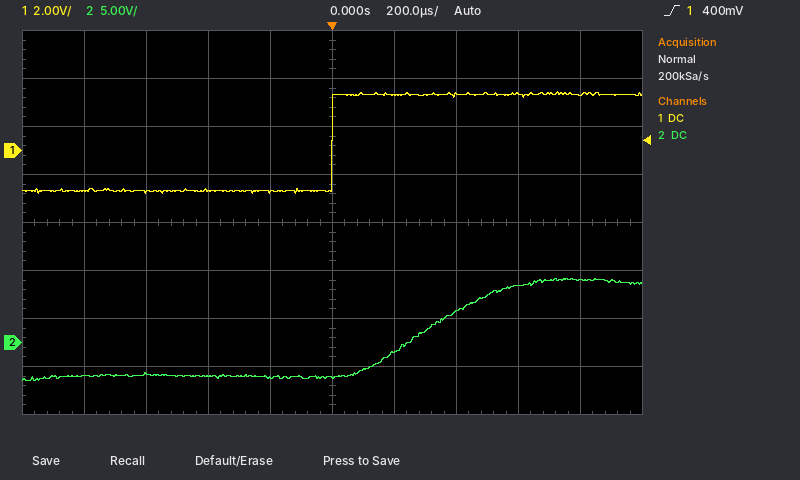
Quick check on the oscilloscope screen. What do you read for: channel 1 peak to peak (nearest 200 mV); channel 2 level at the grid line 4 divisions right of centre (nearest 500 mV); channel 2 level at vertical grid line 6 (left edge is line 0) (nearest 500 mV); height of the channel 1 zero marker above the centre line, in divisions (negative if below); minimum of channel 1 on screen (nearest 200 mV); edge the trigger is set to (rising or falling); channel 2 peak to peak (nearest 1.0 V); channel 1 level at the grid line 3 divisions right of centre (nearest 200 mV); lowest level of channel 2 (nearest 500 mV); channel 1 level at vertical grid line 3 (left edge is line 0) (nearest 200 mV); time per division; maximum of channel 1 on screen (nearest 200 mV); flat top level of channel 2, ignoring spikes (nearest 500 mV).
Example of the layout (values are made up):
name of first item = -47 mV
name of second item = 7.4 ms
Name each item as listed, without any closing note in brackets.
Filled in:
channel 1 peak to peak = 4.2 V
channel 2 level at the grid line 4 divisions right of centre = 6.5 V
channel 2 level at vertical grid line 6 (left edge is line 0) = -1.0 V
height of the channel 1 zero marker above the centre line, in divisions = +1.5 div
minimum of channel 1 on screen = -1.8 V
edge the trigger is set to = rising
channel 2 peak to peak = 11.0 V
channel 1 level at the grid line 3 divisions right of centre = 2.4 V
lowest level of channel 2 = -4.0 V
channel 1 level at vertical grid line 3 (left edge is line 0) = -1.6 V
time per division = 200 µs
maximum of channel 1 on screen = 2.4 V
flat top level of channel 2, ignoring spikes = 6.5 V
